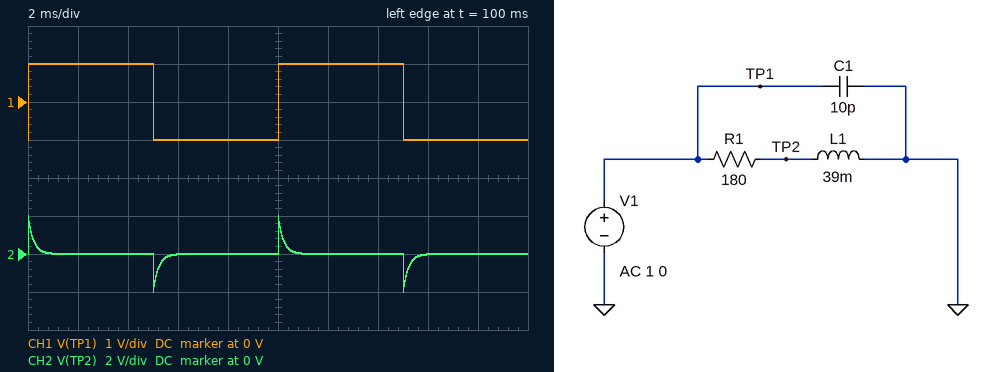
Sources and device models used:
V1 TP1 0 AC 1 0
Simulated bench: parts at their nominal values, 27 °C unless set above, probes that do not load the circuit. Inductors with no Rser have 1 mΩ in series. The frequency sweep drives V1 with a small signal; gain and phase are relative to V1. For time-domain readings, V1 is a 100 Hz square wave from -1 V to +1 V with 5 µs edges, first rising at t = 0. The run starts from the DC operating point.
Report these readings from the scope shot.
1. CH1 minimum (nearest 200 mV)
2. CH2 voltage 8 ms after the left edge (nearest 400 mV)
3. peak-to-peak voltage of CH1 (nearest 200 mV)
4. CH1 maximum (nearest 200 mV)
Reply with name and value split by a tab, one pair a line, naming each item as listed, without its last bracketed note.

CH1 minimum	-1.0 V
CH2 voltage 8 ms after the left edge	0 V
peak-to-peak voltage of CH1	2.0 V
CH1 maximum	1.0 V
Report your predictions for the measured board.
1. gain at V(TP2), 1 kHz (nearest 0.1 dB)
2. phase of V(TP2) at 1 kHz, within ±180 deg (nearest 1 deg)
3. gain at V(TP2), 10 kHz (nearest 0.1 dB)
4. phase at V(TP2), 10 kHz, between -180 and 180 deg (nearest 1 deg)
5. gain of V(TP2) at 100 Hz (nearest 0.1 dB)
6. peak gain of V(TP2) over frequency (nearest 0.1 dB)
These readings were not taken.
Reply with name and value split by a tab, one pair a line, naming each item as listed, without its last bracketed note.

gain at V(TP2), 1 kHz	-1.9 dB
phase of V(TP2) at 1 kHz, within ±180 deg	36 deg
gain at V(TP2), 10 kHz	0 dB
phase at V(TP2), 10 kHz, between -180 and 180 deg	4 deg
gain of V(TP2) at 100 Hz	-17.4 dB
peak gain of V(TP2) over frequency	0 dB
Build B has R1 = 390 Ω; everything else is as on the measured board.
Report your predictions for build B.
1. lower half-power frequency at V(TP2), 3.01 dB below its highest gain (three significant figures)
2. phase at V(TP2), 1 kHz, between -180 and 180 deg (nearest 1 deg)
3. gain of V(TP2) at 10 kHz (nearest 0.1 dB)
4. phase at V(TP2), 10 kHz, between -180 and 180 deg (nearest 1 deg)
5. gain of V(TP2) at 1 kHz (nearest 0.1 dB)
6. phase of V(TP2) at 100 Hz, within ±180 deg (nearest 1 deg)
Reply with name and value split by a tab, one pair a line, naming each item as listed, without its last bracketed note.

lower half-power frequency at V(TP2), 3.01 dB below its highest gain	1.59 kHz
phase at V(TP2), 1 kHz, between -180 and 180 deg	58 deg
gain of V(TP2) at 10 kHz	-0.1 dB
phase at V(TP2), 10 kHz, between -180 and 180 deg	9 deg
gain of V(TP2) at 1 kHz	-5.5 dB
phase of V(TP2) at 100 Hz, within ±180 deg	86 deg
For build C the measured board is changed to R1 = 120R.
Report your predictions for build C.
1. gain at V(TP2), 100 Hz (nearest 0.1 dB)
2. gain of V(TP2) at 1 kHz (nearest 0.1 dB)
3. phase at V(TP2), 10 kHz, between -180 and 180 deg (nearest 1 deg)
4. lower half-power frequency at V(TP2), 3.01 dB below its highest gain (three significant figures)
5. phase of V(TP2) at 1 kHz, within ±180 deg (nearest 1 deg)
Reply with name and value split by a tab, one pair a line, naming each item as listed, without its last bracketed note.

gain at V(TP2), 100 Hz	-14.0 dB
gain of V(TP2) at 1 kHz	-0.9 dB
phase at V(TP2), 10 kHz, between -180 and 180 deg	3 deg
lower half-power frequency at V(TP2), 3.01 dB below its highest gain	490 Hz
phase of V(TP2) at 1 kHz, within ±180 deg	26 deg
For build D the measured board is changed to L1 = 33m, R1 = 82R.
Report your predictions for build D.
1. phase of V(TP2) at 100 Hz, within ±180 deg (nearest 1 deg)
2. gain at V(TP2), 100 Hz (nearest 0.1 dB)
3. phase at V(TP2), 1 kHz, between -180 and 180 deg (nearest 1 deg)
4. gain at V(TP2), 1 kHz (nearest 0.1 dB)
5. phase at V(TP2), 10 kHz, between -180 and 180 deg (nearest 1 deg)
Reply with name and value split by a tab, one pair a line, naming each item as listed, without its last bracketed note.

phase of V(TP2) at 100 Hz, within ±180 deg	76 deg
gain at V(TP2), 100 Hz	-12.2 dB
phase at V(TP2), 1 kHz, between -180 and 180 deg	22 deg
gain at V(TP2), 1 kHz	-0.6 dB
phase at V(TP2), 10 kHz, between -180 and 180 deg	2 deg
